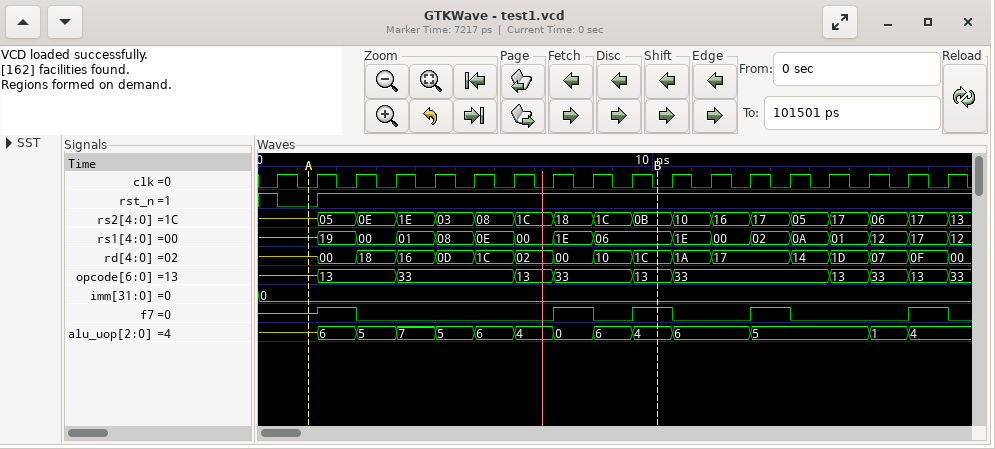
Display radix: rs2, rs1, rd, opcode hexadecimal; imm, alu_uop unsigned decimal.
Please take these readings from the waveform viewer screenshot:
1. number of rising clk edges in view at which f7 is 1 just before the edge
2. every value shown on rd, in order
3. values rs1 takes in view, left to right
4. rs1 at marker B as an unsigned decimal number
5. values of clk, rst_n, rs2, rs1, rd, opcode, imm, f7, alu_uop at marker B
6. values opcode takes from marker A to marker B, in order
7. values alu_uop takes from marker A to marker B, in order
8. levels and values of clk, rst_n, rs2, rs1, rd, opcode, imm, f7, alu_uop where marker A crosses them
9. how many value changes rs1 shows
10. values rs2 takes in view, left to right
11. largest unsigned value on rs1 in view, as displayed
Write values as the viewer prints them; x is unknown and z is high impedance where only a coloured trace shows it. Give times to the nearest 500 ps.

5
z, 00, 18, 16, 0D, 1C, 02, 00, 10, 1C, 1A, 17, 14, 1D, 07, 0F, 00
z, 19, 00, 01, 08, 0E, 00, 1E, 06, 1E, 00, 02, 0A, 01, 12, 17, 12
6
clk=0, rst_n=1, rs2=0B, rs1=06, rd=1C, opcode=13, imm=0, f7=1, alu_uop=4
z, 13, 33, 13, 33, 13
z, 6, 5, 7, 5, 6, 4, 0, 6, 4
clk=0, rst_n=0, rs2=z, rs1=z, rd=z, opcode=z, imm=0, f7=z, alu_uop=z
16
z, 05, 0E, 1E, 03, 08, 1C, 18, 1C, 0B, 10, 16, 17, 05, 17, 06, 17, 13
1E
